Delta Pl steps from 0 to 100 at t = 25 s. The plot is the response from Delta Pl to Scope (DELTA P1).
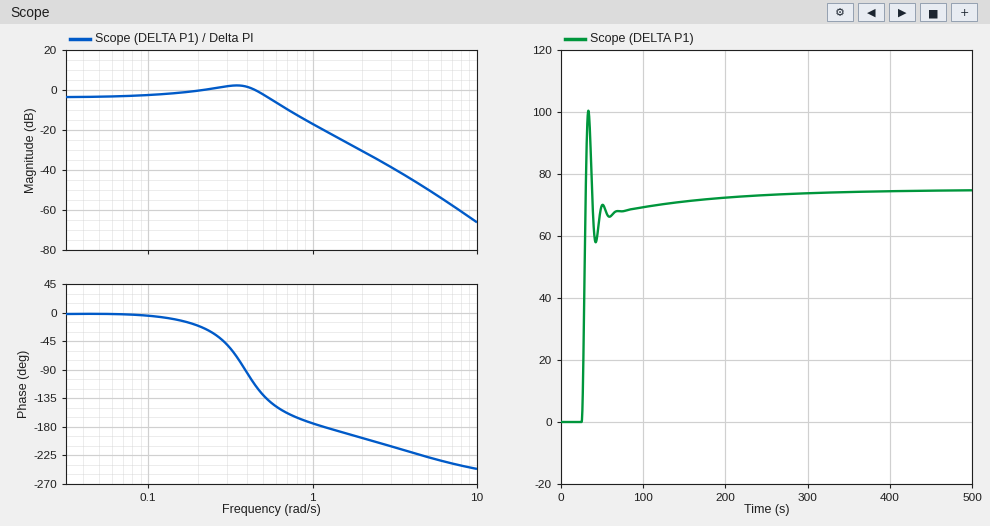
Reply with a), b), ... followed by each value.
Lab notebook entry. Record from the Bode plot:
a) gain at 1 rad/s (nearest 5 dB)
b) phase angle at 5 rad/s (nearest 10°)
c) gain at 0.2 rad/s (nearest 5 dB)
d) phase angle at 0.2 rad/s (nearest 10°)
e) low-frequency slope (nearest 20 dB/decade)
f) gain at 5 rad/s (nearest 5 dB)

a) -15 dB
b) -230°
c) 0 dB
d) -20°
e) 0 dB/decade
f) -50 dB
